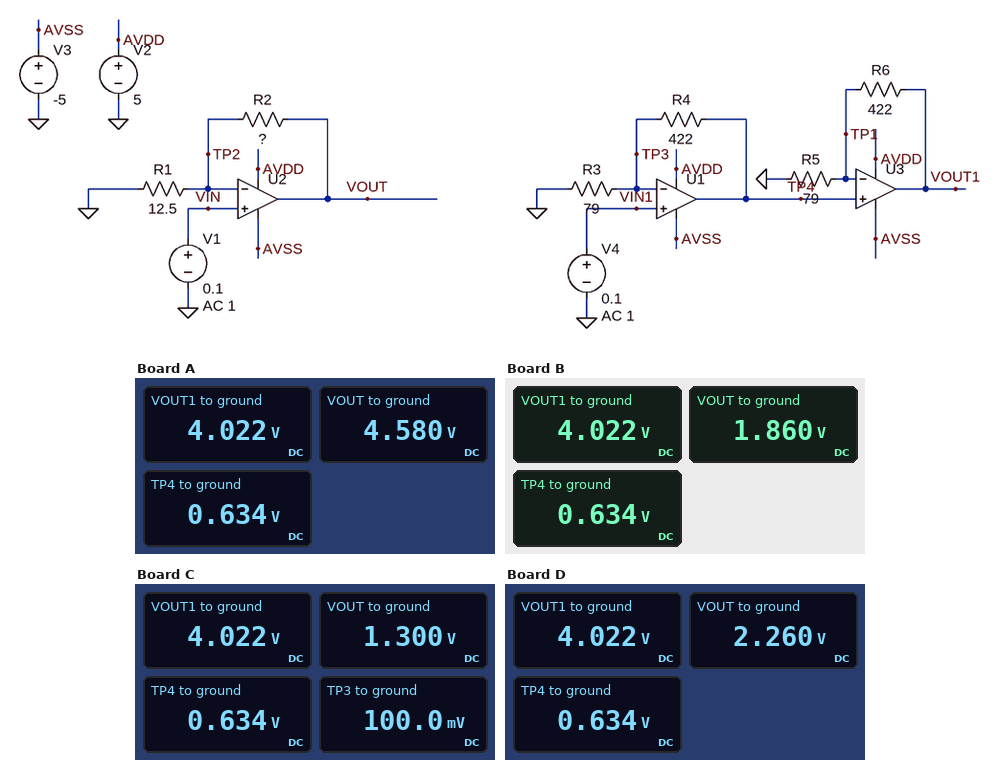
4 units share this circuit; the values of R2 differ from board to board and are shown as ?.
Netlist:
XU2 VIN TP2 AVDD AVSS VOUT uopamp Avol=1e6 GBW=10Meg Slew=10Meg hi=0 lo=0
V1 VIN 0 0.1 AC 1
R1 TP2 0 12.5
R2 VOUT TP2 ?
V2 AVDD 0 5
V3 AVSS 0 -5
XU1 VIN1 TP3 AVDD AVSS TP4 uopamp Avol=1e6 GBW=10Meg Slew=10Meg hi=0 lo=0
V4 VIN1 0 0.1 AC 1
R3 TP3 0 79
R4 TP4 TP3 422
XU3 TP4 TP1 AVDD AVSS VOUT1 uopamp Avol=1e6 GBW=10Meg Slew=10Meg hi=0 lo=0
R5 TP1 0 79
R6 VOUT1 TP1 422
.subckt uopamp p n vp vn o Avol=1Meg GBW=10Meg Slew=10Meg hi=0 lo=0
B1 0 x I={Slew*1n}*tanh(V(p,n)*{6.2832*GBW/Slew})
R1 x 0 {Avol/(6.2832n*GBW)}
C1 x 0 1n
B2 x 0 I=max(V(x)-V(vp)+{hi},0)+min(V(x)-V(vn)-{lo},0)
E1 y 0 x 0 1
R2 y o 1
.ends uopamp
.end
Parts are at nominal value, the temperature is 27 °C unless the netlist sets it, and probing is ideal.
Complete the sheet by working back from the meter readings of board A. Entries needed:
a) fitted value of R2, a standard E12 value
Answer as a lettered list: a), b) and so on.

a) 560 Ω
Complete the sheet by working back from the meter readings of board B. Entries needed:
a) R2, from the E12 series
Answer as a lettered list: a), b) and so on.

a) 220 Ω
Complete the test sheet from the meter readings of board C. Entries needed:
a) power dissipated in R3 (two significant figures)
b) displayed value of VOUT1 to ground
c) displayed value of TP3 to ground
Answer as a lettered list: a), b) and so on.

a) 130 µW
b) 4.022 V
c) 100.0 mV
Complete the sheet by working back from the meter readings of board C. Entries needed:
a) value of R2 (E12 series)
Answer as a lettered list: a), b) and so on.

a) 150 Ω
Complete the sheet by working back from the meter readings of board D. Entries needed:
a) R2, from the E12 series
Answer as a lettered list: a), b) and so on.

a) 270 Ω
